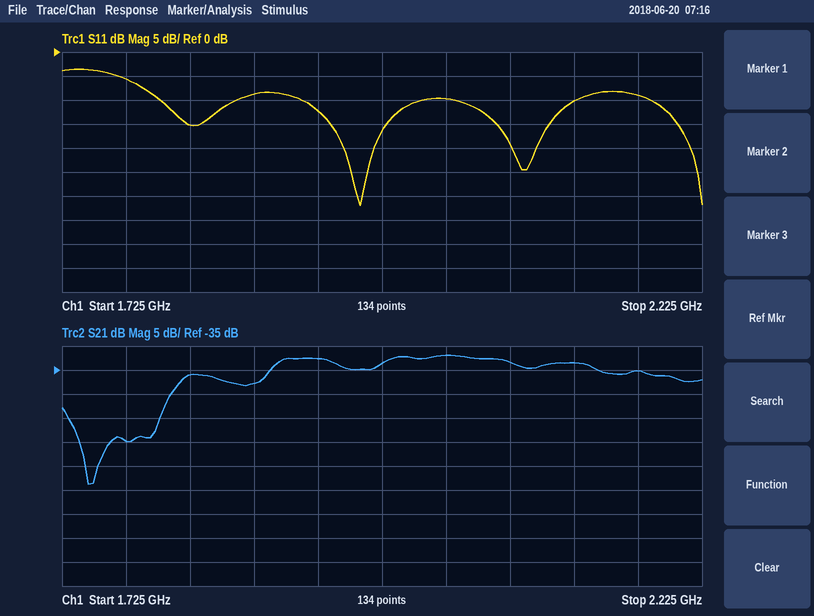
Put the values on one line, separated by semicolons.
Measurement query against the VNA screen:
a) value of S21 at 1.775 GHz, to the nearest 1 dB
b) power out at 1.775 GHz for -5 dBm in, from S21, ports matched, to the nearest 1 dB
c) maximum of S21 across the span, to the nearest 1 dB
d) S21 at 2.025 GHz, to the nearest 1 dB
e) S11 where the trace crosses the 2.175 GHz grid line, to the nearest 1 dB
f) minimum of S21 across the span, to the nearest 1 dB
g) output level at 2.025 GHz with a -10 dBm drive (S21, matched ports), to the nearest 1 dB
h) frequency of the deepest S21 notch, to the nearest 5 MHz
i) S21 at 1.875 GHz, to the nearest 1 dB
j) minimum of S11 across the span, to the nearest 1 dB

-50 dB; -55 dBm; -32 dB; -32 dB; -9 dB; -59 dB; -42 dBm; 1.745 GHz; -38 dB; -32 dB
